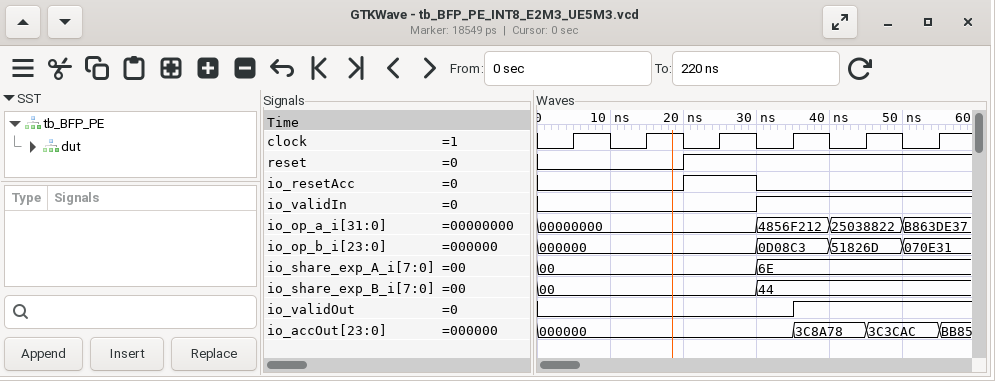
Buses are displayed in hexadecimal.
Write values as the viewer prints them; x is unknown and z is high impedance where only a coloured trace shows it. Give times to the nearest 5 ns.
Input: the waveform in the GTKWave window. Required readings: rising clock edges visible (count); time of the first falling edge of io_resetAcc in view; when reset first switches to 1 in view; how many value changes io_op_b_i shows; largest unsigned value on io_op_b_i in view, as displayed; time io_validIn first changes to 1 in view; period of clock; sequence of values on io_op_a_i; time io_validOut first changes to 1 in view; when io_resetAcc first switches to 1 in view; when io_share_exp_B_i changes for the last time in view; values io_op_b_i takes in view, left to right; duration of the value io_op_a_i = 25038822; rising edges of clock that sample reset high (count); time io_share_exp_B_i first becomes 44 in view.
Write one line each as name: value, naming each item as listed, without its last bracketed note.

rising clock edges visible: 6
time of the first falling edge of io_resetAcc in view: 30 ns
when reset first switches to 1 in view: 20 ns
how many value changes io_op_b_i shows: 3
largest unsigned value on io_op_b_i in view, as displayed: 51826D
time io_validIn first changes to 1 in view: 30 ns
period of clock: 10 ns
sequence of values on io_op_a_i: 00000000, 4856F212, 25038822, B863DE37
time io_validOut first changes to 1 in view: 35 ns
when io_resetAcc first switches to 1 in view: 20 ns
when io_share_exp_B_i changes for the last time in view: 30 ns
values io_op_b_i takes in view, left to right: 000000, 0D08C3, 51826D, 070E31
duration of the value io_op_a_i = 25038822: 10 ns
rising edges of clock that sample reset high: 4
time io_share_exp_B_i first becomes 44 in view: 30 ns
